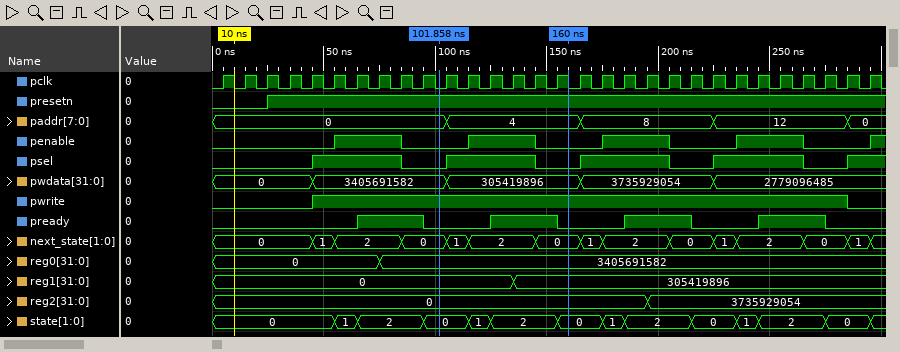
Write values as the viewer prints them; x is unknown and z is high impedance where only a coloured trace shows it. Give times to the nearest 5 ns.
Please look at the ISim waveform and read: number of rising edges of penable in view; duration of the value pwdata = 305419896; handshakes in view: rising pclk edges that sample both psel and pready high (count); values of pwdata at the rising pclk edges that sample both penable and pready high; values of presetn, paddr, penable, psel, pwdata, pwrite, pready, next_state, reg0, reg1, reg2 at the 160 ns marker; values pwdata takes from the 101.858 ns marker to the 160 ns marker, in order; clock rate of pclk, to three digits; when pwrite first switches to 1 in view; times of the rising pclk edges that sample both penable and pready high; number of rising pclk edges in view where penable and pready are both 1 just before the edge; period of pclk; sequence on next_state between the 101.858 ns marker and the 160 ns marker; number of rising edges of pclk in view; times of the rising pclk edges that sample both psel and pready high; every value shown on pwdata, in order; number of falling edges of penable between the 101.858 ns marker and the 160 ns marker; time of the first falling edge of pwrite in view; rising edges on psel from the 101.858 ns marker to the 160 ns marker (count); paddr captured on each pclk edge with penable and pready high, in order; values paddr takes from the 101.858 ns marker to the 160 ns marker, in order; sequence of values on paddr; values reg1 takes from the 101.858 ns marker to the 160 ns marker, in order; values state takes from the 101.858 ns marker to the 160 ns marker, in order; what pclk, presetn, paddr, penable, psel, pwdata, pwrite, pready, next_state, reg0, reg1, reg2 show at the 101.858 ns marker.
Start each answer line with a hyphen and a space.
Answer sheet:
- 5
- 60 ns
- 8
- 3405691582, 3405691582, 305419896, 305419896, 3735929054, 3735929054, 2779096485, 2779096485
- presetn=1, paddr=4, penable=0, psel=0, pwdata=305419896, pwrite=1, pready=0, next_state=0, reg0=3405691582, reg1=305419896, reg2=0
- 3405691582, 305419896
- 100 MHz
- 45 ns
- 75 ns, 85 ns, 135 ns, 145 ns, 195 ns, 205 ns, 255 ns, 265 ns
- 8
- 10 ns
- 0, 1, 2, 0
- 30
- 75 ns, 85 ns, 135 ns, 145 ns, 195 ns, 205 ns, 255 ns, 265 ns
- 0, 3405691582, 305419896, 3735929054, 2779096485
- 1
- 285 ns
- 1
- 0, 0, 4, 4, 8, 8, 12, 12
- 0, 4
- 0, 4, 8, 12, 0
- 0, 305419896
- 0, 1, 2, 0
- pclk=0, presetn=1, paddr=0, penable=0, psel=0, pwdata=3405691582, pwrite=1, pready=0, next_state=0, reg0=3405691582, reg1=0, reg2=0
